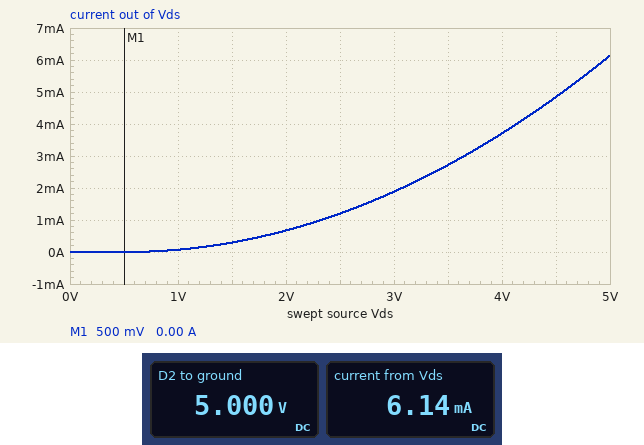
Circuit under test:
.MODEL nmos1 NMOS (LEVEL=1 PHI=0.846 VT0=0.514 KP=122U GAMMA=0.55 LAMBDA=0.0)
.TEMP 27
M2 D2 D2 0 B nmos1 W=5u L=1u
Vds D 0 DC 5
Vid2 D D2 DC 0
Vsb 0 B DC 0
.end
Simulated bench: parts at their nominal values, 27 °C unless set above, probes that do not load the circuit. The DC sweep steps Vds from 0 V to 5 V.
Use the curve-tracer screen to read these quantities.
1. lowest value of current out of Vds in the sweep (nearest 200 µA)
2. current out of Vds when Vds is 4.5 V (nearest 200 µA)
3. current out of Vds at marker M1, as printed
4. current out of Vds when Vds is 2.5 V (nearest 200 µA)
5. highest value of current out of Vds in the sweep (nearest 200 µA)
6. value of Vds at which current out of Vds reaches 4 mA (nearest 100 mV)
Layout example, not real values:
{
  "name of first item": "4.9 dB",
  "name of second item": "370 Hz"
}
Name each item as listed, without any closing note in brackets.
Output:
{
  "lowest value of current out of Vds in the sweep": "0 A",
  "current out of Vds when Vds is 4.5 V": "4.8 mA",
  "current out of Vds at marker M1, as printed": "0.00 A",
  "current out of Vds when Vds is 2.5 V": "1.2 mA",
  "highest value of current out of Vds in the sweep": "6.2 mA",
  "value of Vds at which current out of Vds reaches 4 mA": "4.1 V"
}
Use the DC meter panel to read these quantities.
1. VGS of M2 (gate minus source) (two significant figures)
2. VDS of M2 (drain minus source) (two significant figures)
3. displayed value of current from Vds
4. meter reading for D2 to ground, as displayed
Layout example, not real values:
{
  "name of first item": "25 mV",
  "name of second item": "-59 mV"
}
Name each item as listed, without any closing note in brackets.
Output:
{
  "VGS of M2 (gate minus source)": "5.0 V",
  "VDS of M2 (drain minus source)": "5.0 V",
  "displayed value of current from Vds": "6.14 mA",
  "meter reading for D2 to ground, as displayed": "5.000 V"
}
